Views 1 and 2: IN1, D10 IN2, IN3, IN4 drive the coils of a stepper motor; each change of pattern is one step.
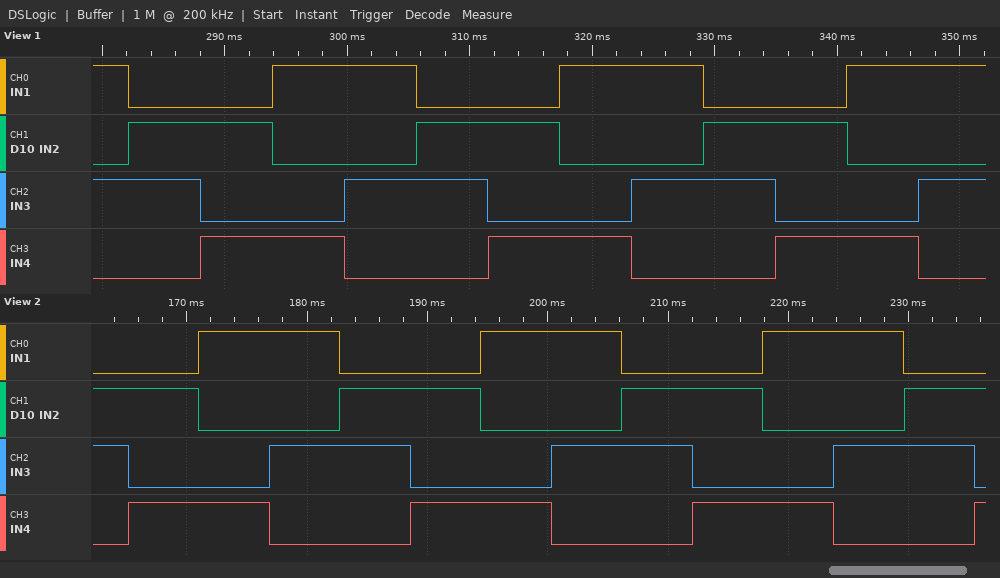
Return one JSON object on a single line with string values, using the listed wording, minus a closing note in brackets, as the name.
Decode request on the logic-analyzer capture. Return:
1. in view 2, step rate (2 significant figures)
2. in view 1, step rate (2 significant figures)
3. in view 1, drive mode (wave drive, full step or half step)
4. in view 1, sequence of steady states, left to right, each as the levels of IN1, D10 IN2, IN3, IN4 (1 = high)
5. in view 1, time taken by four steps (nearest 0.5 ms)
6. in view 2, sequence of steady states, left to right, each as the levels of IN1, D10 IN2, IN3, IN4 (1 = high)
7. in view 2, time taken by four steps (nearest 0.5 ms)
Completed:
{"in view 2, step rate": "170 steps/s", "in view 1, step rate": "170 steps/s", "in view 1, drive mode": "full step", "in view 1, sequence of steady states, left to right, each as the levels of IN1, D10 IN2, IN3, IN4": "1010 0110 0101 1001 1010 0110 0101 1001 1010 0110 0101 1001 1010", "in view 1, time taken by four steps": "23.5 ms", "in view 2, sequence of steady states, left to right, each as the levels of IN1, D10 IN2, IN3, IN4": "0110 0101 1001 1010 0110 0101 1001 1010 0110 0101 1001 1010 0110 0101", "in view 2, time taken by four steps": "23.5 ms"}
